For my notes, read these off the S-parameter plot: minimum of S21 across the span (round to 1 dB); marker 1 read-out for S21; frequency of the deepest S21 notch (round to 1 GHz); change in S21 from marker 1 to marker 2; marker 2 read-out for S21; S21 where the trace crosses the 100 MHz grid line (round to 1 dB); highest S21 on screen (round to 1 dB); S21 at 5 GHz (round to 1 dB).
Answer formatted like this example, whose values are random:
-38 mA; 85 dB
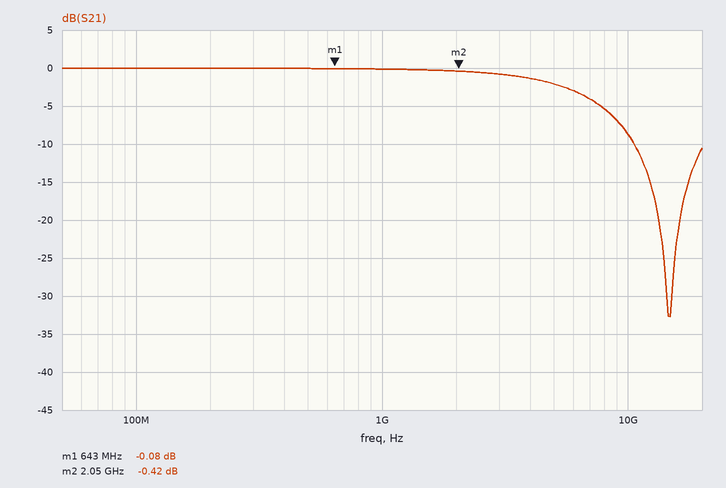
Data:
-33 dB; -0.08 dB; 15 GHz; -0.34 dB; -0.42 dB; 0 dB; 0 dB; -2 dB
